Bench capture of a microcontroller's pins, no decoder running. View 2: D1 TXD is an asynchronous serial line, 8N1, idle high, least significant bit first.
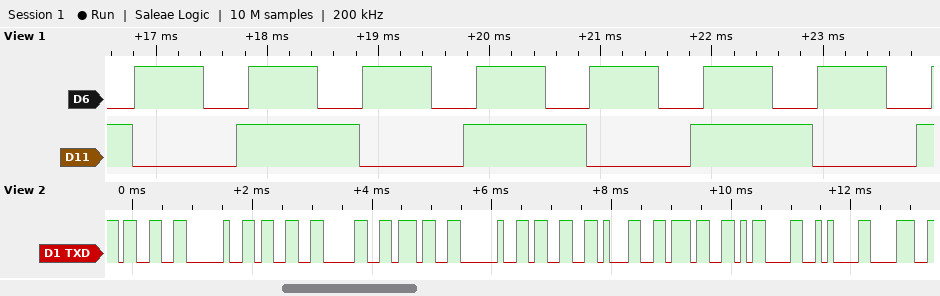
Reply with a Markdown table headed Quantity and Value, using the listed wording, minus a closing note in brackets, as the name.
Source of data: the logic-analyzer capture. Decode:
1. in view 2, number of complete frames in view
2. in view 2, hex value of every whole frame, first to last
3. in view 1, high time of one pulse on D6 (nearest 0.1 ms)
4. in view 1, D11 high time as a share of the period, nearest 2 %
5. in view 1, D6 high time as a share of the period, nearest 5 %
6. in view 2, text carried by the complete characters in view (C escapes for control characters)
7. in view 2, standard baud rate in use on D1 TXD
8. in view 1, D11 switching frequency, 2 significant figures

| Quantity | Value |
|---|---|
| in view 2, number of complete frames in view | 12 |
| in view 2, hex value of every whole frame, first to last | 33 20 33 30 37 20 33 31 37 0D 0A 38 |
| in view 1, high time of one pulse on D6 | 0.6 ms |
| in view 1, D11 high time as a share of the period, nearest 2 % | 54 % |
| in view 1, D6 high time as a share of the period, nearest 5 % | 60 % |
| in view 2, text carried by the complete characters in view | "3 307 317\r\n8" |
| in view 2, standard baud rate in use on D1 TXD | 9600 baud |
| in view 1, D11 switching frequency, 2 significant figures | 490 Hz |
